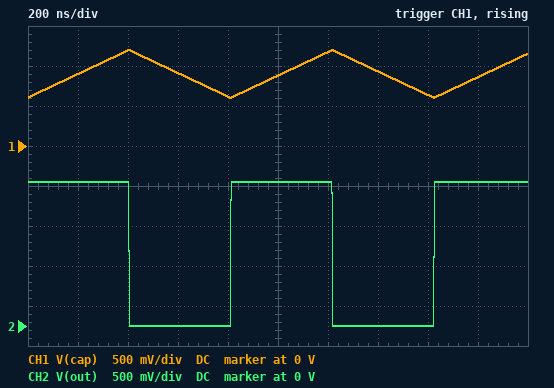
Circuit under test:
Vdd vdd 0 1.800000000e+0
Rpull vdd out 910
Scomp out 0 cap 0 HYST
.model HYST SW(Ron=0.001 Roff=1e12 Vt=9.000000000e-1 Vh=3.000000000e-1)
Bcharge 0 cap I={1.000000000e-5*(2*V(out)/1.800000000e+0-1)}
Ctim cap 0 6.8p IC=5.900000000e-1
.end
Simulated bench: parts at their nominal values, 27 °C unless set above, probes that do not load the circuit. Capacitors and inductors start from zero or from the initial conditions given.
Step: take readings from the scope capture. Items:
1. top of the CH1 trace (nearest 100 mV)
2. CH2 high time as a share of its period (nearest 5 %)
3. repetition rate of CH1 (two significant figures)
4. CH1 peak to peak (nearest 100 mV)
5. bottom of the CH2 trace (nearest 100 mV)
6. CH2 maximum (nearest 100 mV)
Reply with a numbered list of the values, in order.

1. 1.2 V
2. 50 %
3. 1.2 MHz
4. 600 mV
5. 0 V
6. 1.8 V
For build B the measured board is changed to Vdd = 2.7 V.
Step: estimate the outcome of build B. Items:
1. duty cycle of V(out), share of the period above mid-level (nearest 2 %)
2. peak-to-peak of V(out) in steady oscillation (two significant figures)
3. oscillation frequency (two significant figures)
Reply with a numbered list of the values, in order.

1. 34 %
2. 2.7 V
3. 1.6 MHz
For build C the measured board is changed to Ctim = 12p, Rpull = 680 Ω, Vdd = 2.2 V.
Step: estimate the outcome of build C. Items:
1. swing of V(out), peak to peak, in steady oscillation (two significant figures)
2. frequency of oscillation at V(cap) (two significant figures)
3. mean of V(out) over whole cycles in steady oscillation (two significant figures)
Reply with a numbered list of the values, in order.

1. 2.2 V
2. 820 kHz
3. 900 mV
